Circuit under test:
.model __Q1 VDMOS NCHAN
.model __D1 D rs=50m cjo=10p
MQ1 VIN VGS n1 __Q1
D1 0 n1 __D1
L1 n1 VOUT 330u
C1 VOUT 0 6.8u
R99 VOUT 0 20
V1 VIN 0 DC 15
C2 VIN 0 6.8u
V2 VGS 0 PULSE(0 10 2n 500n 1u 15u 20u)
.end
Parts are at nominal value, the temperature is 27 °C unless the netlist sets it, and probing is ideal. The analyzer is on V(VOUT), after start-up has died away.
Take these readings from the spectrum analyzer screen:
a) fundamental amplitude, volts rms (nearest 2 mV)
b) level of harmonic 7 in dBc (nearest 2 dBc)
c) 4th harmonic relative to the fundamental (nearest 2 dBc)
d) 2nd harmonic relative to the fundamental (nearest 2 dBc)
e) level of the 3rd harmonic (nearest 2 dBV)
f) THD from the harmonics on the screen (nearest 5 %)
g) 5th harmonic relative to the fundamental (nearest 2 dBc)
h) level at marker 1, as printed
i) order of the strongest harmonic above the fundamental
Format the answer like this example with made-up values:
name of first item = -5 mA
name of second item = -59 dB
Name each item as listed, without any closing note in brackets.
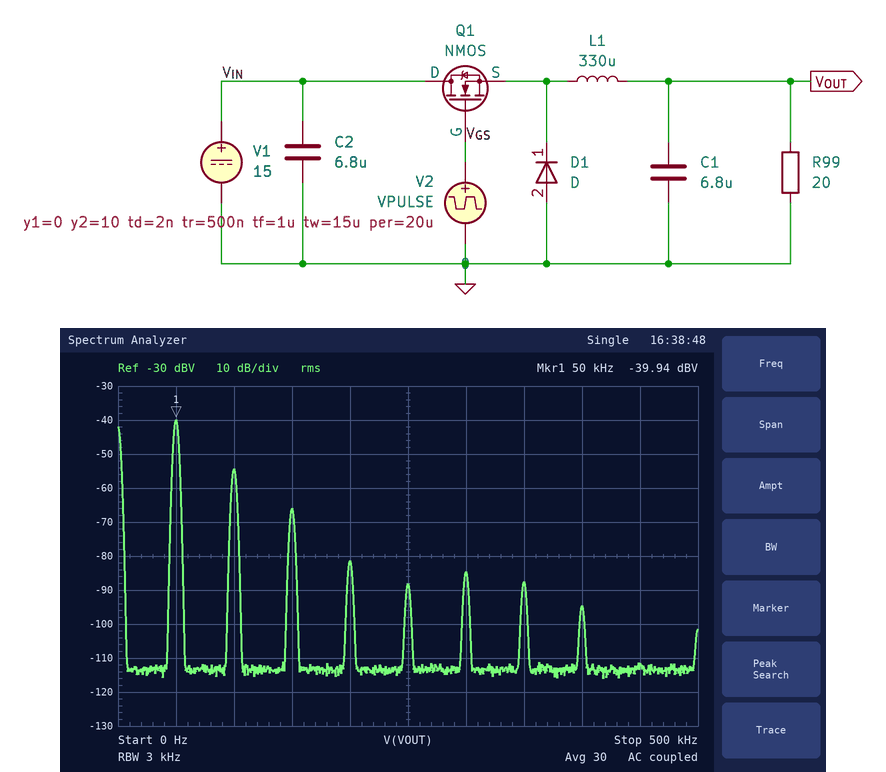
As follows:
fundamental amplitude, volts rms = 10 mV
level of harmonic 7 in dBc = -48 dBc
4th harmonic relative to the fundamental = -42 dBc
2nd harmonic relative to the fundamental = -14 dBc
level of the 3rd harmonic = -66 dBV
THD from the harmonics on the screen = 20 %
5th harmonic relative to the fundamental = -48 dBc
level at marker 1, as printed = -39.94 dBV
order of the strongest harmonic above the fundamental = 2
